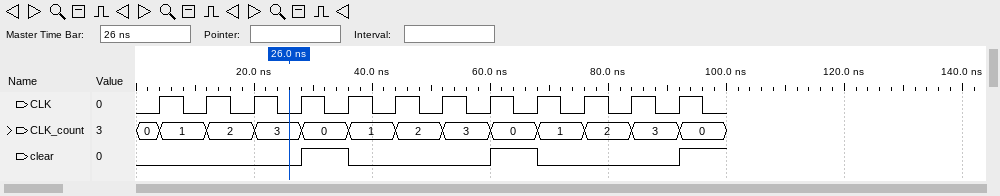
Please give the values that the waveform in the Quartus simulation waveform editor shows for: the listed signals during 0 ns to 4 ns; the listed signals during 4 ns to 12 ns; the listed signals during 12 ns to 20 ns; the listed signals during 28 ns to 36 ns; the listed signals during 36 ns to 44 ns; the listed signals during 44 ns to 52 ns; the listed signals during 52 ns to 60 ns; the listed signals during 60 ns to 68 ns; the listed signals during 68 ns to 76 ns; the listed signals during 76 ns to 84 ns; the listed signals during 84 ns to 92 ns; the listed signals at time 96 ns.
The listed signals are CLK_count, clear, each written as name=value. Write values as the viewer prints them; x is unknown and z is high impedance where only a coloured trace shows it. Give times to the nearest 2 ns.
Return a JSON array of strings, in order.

["CLK_count=0, clear=0", "CLK_count=1, clear=0", "CLK_count=2, clear=0", "CLK_count=0, clear=1", "CLK_count=1, clear=0", "CLK_count=2, clear=0", "CLK_count=3, clear=0", "CLK_count=0, clear=1", "CLK_count=1, clear=0", "CLK_count=2, clear=0", "CLK_count=3, clear=0", "CLK_count=0, clear=1"]
